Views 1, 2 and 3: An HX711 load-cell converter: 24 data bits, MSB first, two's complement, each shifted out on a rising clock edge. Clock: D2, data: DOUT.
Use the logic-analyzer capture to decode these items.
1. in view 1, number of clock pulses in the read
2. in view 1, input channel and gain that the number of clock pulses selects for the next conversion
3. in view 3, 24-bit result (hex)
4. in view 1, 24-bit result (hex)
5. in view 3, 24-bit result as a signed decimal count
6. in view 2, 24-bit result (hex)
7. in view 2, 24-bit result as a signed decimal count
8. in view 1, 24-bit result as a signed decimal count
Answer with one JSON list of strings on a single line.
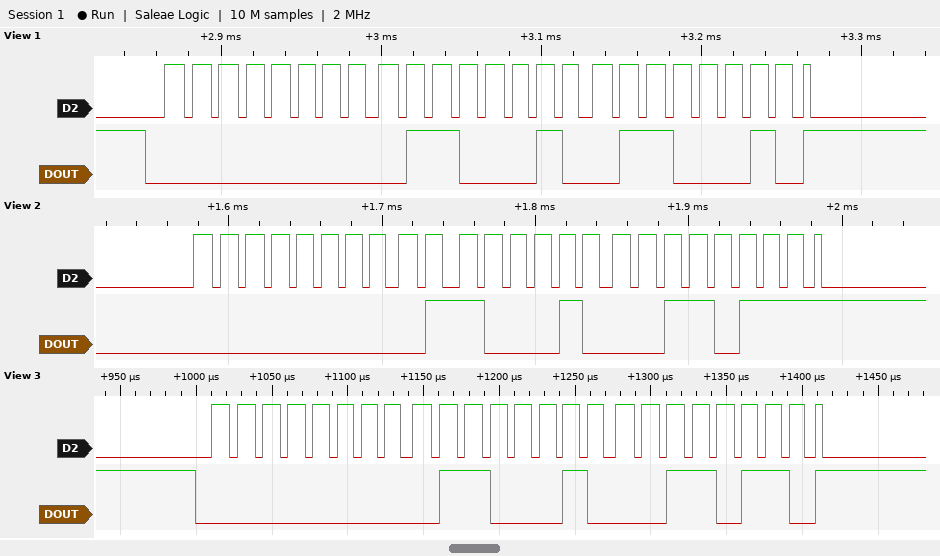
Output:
["25", "channel A, gain 128", "0x006236", "0x006262", "25142", "0x006237", "25143", "25186"]
